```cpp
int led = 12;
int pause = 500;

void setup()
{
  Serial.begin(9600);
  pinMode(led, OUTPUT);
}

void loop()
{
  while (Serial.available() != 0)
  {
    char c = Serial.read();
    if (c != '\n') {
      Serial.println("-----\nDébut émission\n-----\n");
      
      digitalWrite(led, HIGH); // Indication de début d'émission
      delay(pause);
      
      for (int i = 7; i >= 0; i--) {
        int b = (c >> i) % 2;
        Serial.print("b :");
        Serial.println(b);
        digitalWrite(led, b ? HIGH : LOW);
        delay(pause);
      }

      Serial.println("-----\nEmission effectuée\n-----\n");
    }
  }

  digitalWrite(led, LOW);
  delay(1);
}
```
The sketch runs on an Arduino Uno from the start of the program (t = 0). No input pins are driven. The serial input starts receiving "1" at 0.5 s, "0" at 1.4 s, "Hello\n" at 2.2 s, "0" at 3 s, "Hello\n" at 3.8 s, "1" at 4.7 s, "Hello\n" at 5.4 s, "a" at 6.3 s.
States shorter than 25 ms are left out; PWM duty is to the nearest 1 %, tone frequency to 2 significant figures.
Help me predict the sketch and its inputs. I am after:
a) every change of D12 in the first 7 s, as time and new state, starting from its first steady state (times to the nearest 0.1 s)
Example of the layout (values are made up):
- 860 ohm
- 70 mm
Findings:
- 0 s low; 0.5 s high; 1 s low; 2 s high; 3 s low; 4.5 s high; 5.5 s low; 6.5 s high
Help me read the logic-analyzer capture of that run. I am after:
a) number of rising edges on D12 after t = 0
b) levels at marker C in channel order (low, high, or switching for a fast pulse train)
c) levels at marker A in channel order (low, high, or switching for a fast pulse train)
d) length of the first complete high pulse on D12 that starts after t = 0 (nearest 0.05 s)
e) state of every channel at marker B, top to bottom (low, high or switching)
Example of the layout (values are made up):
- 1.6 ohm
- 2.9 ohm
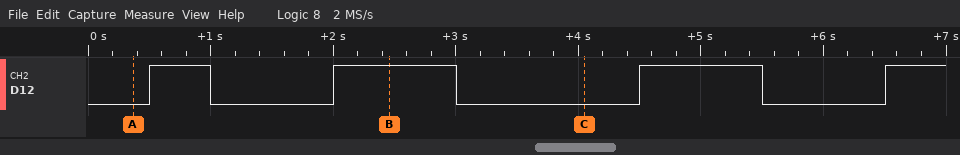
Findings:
- 4
- D12 low
- D12 low
- 0.50 s
- D12 high
